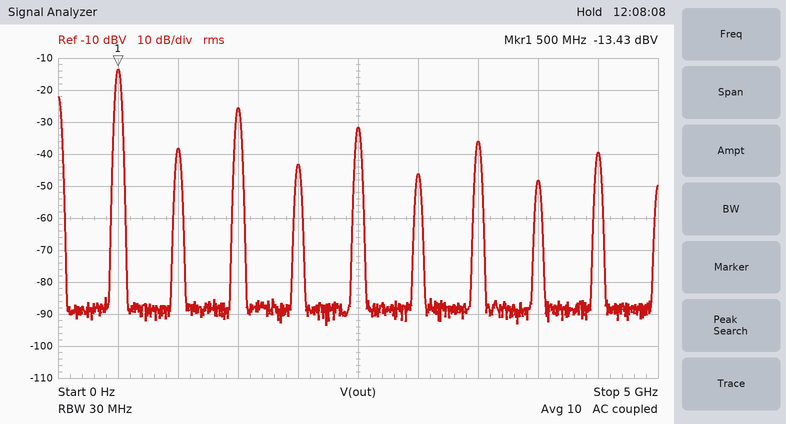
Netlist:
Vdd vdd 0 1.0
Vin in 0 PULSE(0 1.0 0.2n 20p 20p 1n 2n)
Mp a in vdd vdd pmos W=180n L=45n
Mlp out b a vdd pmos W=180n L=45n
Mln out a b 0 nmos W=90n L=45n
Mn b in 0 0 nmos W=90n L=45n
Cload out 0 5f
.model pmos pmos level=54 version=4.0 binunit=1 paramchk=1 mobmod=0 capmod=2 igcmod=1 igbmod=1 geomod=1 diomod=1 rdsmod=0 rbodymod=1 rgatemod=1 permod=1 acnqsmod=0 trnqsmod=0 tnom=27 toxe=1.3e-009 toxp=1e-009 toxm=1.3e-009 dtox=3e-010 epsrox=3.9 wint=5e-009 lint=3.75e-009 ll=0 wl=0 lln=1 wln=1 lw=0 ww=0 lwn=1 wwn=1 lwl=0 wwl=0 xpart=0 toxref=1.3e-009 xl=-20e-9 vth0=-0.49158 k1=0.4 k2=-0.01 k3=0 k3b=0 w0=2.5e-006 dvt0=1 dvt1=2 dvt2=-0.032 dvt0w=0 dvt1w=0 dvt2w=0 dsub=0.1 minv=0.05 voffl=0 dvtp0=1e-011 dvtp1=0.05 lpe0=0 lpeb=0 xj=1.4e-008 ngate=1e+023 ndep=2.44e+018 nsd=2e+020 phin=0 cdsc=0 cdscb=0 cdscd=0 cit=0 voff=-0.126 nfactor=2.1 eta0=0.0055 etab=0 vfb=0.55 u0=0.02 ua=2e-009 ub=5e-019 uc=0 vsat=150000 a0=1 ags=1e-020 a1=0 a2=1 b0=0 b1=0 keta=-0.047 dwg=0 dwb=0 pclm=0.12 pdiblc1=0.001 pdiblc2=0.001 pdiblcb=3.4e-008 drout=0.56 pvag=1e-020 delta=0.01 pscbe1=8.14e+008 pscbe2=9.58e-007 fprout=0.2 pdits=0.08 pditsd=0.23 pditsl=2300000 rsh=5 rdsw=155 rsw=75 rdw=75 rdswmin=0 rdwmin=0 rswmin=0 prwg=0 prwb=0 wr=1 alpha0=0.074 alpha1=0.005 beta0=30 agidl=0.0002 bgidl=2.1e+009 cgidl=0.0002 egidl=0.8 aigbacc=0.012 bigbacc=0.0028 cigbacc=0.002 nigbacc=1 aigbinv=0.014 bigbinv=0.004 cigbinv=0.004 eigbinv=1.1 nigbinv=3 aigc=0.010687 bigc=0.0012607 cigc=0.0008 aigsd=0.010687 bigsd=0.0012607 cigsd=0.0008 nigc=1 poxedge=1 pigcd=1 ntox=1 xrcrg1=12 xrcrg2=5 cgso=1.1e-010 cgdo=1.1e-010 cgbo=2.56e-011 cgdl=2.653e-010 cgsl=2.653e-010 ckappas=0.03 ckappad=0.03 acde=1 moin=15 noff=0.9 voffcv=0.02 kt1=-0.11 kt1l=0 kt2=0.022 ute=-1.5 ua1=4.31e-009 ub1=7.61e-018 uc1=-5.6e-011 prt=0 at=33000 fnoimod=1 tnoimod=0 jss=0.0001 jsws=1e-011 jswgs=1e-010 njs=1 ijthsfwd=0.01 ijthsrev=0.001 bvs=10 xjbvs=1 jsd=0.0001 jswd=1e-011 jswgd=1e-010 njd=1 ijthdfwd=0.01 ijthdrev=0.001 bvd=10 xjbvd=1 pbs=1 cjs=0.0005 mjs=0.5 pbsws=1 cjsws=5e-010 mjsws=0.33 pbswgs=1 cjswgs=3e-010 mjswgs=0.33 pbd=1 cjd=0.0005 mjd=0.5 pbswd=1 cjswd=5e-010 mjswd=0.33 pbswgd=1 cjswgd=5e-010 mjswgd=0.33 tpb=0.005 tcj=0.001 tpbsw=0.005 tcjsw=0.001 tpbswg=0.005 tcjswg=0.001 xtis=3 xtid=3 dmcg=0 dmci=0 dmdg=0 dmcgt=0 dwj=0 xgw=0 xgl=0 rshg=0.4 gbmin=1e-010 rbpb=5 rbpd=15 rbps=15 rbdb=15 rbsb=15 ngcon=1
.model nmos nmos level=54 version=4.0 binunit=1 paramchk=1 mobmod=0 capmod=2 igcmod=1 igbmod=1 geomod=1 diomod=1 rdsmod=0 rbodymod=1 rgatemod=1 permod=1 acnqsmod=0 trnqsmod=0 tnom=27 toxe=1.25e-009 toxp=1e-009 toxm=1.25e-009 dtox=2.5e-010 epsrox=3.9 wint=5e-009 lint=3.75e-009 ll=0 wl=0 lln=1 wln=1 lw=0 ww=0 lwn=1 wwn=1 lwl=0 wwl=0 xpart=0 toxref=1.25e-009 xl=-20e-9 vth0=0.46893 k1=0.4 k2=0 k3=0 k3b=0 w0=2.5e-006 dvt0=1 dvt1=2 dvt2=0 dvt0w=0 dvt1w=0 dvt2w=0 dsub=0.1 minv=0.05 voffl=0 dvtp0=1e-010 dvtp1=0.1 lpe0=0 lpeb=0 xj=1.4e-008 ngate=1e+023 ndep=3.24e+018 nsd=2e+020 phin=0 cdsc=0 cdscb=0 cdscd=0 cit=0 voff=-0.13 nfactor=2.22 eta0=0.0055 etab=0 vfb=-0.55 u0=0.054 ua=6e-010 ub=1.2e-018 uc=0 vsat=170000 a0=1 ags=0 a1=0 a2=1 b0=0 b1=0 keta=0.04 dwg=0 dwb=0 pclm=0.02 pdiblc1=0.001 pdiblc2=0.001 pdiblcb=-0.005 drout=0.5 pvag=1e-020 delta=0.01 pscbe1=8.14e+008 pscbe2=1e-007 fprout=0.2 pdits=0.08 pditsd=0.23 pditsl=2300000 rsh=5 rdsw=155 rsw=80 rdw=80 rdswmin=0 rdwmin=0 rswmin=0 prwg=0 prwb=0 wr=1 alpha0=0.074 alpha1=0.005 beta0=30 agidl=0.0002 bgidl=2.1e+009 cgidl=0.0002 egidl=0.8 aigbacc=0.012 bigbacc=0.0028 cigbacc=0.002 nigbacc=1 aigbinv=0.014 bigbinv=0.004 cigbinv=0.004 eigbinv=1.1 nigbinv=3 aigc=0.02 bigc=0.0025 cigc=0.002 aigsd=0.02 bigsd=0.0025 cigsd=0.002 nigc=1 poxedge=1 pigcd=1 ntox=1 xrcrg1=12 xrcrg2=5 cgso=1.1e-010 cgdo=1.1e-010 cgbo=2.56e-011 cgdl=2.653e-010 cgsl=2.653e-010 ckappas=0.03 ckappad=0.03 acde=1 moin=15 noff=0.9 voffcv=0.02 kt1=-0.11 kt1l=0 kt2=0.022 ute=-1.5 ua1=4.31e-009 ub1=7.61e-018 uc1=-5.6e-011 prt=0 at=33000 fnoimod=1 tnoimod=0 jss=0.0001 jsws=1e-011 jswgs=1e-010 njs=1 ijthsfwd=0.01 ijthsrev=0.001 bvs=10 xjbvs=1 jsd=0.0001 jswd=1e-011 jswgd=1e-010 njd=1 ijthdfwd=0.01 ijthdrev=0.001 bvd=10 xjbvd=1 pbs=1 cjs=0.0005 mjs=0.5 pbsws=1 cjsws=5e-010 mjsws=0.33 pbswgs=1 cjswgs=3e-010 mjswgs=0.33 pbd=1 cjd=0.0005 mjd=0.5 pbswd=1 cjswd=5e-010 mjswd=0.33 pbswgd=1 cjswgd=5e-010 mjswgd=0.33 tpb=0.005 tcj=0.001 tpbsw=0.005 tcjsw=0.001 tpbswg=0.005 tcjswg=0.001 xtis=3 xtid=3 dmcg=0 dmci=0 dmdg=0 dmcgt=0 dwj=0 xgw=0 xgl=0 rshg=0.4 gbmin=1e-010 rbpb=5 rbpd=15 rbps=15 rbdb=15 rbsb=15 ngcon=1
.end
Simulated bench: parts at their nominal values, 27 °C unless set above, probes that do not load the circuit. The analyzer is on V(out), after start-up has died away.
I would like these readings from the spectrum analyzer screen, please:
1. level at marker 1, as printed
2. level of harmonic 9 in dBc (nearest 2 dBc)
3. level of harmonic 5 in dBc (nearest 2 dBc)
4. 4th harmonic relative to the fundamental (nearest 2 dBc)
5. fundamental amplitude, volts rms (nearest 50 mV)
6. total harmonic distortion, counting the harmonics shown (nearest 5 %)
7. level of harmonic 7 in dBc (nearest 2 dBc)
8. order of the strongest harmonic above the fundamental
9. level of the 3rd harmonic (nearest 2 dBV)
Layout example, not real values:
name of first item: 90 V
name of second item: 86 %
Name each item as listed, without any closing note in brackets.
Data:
level at marker 1, as printed: -13.43 dBV
level of harmonic 9 in dBc: -26 dBc
level of harmonic 5 in dBc: -18 dBc
4th harmonic relative to the fundamental: -30 dBc
fundamental amplitude, volts rms: 200 mV
total harmonic distortion, counting the harmonics shown: 30 %
level of harmonic 7 in dBc: -22 dBc
order of the strongest harmonic above the fundamental: 3
level of the 3rd harmonic: -26 dBV
